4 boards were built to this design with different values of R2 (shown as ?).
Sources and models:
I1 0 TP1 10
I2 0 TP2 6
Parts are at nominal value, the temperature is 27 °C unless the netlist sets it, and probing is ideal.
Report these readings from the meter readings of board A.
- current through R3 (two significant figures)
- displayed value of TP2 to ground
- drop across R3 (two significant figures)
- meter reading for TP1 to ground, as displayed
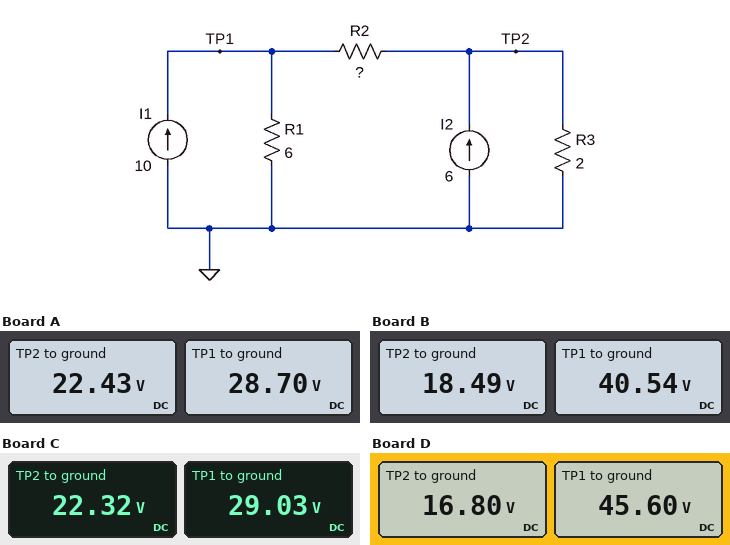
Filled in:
11 A
22.43 V
22 V
28.70 V
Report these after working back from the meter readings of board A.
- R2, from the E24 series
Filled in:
1.2 Ω
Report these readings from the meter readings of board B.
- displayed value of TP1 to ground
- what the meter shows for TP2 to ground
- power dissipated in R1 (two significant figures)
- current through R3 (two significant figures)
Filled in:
40.54 V
18.49 V
270 W
9.2 A
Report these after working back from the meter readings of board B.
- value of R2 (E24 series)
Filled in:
6.8 Ω
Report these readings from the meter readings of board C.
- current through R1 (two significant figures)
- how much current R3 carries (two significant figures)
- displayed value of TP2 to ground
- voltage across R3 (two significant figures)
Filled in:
4.8 A
11 A
22.32 V
22 V
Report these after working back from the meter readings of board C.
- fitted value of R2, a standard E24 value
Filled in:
1.3 Ω
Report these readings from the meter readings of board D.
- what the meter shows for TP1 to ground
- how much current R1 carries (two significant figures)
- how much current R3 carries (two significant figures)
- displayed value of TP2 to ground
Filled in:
45.60 V
7.6 A
8.4 A
16.80 V
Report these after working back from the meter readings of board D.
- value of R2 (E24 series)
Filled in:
12 Ω
